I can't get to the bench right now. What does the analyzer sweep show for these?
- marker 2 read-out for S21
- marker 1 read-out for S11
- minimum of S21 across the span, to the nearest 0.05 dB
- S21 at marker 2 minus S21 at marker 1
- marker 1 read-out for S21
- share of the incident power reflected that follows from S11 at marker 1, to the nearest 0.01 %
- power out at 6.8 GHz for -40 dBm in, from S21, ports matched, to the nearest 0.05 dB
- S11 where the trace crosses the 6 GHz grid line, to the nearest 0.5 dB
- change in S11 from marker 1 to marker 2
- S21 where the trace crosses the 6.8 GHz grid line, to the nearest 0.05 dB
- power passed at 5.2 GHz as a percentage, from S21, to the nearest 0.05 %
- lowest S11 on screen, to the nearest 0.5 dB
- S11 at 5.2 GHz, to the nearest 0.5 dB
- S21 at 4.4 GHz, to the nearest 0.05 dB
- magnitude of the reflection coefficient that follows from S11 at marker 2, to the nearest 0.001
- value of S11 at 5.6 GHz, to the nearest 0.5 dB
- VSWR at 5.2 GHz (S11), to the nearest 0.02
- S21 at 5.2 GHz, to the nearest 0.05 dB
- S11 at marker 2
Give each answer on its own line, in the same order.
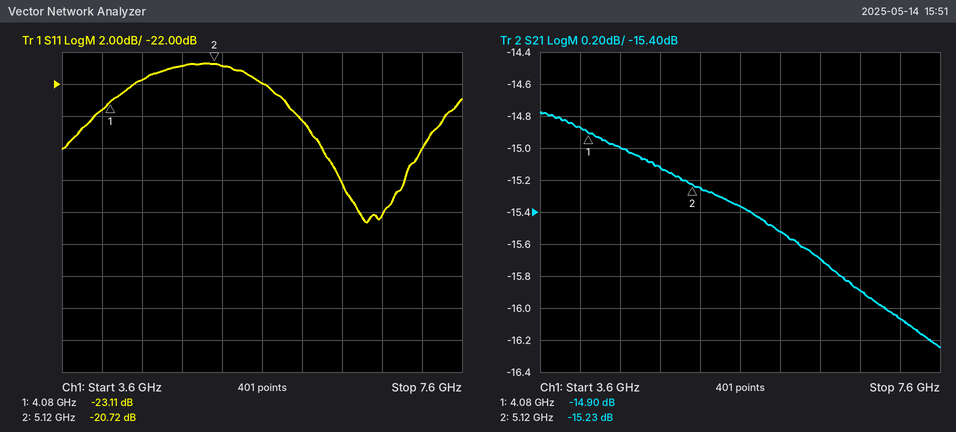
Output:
-15.23 dB
-23.11 dB
-16.25 dB
-0.33 dB
-14.90 dB
0.49 %
-55.90 dBm
-24.5 dB
2.39 dB
-15.90 dB
3.00 %
-30.5 dB
-21.0 dB
-15.00 dB
0.092
-22.0 dB
1.20
-15.25 dB
-20.72 dB
